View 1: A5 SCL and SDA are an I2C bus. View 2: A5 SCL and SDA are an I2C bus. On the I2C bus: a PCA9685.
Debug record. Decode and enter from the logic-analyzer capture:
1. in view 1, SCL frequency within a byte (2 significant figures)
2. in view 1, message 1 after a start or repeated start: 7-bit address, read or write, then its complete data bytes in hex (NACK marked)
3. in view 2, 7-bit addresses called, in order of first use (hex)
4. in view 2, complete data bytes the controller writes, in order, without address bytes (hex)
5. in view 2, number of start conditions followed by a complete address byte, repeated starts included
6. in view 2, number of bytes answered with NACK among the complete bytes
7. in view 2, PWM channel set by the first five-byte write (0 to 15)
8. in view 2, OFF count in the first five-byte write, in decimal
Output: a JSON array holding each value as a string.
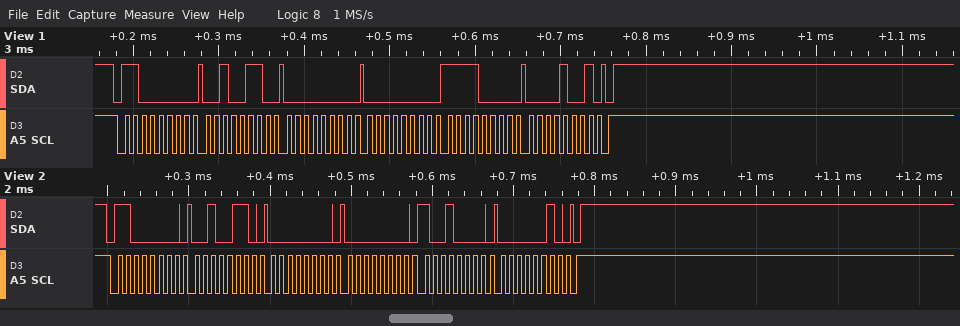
["100 kHz", "0x60 write: 26 00 00 F0 09", "0x60", "26 00 00 90 02", "1", "0", "8", "656"]
